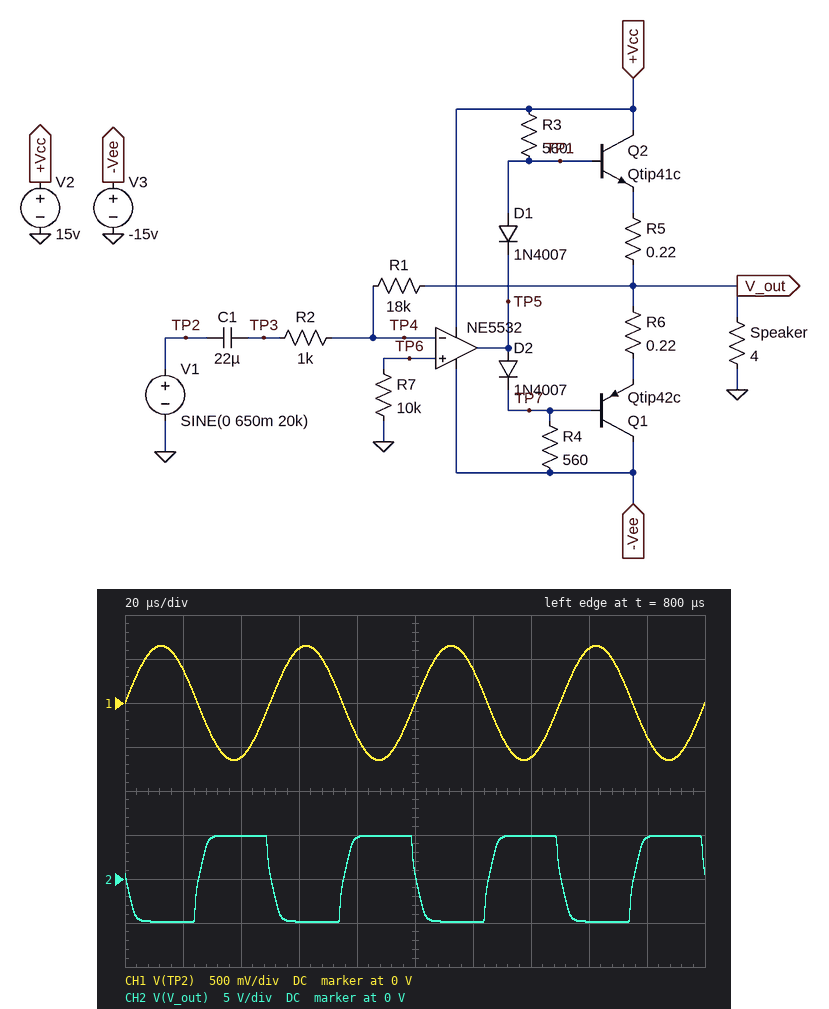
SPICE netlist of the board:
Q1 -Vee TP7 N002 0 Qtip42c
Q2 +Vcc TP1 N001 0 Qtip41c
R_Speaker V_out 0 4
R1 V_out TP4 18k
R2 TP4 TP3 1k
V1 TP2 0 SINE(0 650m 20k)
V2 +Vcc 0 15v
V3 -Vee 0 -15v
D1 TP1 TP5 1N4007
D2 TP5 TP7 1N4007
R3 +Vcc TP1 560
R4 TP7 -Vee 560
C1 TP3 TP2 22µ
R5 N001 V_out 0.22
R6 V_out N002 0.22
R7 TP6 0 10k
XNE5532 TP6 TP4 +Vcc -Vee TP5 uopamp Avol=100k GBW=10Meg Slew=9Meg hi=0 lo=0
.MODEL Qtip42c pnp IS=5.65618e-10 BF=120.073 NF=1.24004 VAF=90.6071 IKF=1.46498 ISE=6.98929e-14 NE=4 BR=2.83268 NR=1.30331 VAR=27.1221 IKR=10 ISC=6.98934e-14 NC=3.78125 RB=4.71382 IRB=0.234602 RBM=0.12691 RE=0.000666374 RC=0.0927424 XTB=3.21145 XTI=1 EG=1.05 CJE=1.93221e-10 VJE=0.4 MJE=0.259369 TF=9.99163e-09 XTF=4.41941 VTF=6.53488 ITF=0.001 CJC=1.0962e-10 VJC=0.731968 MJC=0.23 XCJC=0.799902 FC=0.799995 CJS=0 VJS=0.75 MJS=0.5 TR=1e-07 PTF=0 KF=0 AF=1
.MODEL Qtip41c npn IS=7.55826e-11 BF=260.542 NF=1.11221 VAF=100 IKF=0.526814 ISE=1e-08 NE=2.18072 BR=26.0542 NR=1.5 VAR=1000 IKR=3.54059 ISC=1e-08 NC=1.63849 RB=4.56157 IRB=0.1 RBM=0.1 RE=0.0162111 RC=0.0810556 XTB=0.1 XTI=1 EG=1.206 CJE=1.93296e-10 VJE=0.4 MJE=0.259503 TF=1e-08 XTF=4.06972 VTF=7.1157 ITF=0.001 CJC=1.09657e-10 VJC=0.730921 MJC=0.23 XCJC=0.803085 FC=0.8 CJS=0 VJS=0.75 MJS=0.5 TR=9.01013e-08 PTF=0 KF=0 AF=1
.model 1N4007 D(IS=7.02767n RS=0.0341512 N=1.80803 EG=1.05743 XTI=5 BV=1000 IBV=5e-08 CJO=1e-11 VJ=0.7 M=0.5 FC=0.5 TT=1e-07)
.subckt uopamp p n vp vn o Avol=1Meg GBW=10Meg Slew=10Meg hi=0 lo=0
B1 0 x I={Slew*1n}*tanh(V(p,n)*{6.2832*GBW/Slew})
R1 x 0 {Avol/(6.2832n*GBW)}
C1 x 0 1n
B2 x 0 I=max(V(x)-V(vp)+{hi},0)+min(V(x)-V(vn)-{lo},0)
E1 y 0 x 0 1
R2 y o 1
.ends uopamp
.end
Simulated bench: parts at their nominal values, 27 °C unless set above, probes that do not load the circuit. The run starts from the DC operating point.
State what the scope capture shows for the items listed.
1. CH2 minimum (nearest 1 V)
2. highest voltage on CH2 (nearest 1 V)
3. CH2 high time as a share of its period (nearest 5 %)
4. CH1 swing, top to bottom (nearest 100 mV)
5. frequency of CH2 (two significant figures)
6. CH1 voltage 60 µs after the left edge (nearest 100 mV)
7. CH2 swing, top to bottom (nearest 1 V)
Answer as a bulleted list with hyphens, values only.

- -5 V
- 5 V
- 50 %
- 1.3 V
- 20 kHz
- 600 mV
- 10 V
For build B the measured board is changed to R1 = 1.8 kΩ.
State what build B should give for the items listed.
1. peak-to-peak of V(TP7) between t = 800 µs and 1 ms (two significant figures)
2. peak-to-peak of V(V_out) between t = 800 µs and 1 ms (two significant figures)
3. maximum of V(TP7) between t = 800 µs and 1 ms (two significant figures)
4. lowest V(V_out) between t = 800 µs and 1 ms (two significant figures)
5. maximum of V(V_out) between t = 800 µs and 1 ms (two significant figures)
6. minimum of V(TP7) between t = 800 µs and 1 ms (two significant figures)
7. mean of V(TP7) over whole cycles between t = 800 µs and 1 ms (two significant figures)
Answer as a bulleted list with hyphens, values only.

- 2.5 V
- 2.3 V
- 530 mV
- -1.2 V
- 1.2 V
- -1.9 V
- -700 mV
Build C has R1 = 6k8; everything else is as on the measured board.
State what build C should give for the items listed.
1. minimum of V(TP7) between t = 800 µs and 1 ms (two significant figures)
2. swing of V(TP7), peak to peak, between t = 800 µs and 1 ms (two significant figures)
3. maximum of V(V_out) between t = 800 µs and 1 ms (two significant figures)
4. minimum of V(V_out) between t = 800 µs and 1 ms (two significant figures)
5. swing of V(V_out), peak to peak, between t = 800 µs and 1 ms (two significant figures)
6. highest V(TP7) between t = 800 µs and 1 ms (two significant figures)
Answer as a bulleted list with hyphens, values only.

- -5.4 V
- 9.5 V
- 4.4 V
- -4.4 V
- 8.8 V
- 4.1 V
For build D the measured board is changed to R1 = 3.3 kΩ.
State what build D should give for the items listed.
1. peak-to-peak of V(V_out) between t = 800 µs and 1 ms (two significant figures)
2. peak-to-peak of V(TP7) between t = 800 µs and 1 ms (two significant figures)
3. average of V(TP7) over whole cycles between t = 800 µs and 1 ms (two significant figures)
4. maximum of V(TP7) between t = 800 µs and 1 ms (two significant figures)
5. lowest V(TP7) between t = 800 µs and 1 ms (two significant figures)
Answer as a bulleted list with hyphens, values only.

- 4.3 V
- 4.5 V
- -700 mV
- 1.6 V
- -3.0 V
